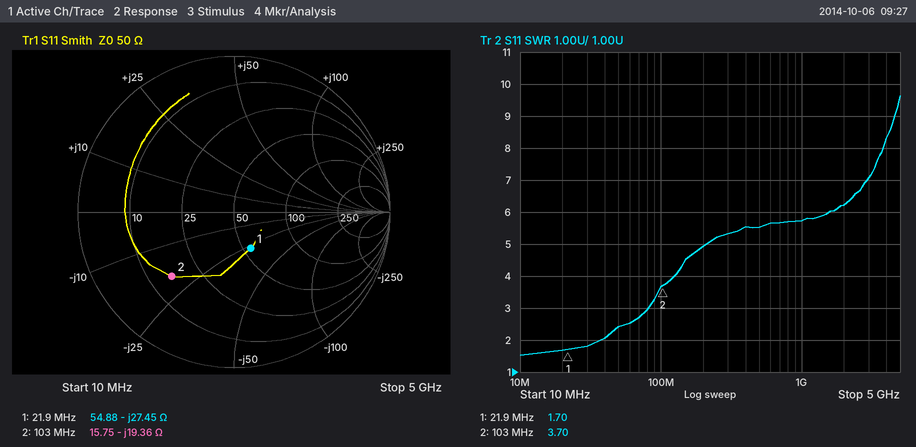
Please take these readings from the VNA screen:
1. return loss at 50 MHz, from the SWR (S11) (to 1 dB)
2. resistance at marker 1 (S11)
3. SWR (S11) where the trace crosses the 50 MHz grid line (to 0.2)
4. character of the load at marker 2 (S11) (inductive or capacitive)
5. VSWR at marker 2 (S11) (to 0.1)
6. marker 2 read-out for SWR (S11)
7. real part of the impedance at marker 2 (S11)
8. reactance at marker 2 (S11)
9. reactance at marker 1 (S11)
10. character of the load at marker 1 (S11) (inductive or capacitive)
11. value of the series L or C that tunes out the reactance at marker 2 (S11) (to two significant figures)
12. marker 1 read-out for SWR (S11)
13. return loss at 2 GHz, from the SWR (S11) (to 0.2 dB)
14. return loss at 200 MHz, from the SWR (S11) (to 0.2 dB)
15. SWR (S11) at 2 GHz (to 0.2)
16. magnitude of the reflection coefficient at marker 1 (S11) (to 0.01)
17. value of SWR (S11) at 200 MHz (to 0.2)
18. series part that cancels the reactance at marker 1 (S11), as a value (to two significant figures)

8 dB
54.88 Ω
2.4
capacitive
3.7
3.70
15.75 Ω
-19.36 Ω
-27.45 Ω
capacitive
30 nH
1.70
2.8 dB
3.6 dB
6.2
0.26
5.0
200 nH
